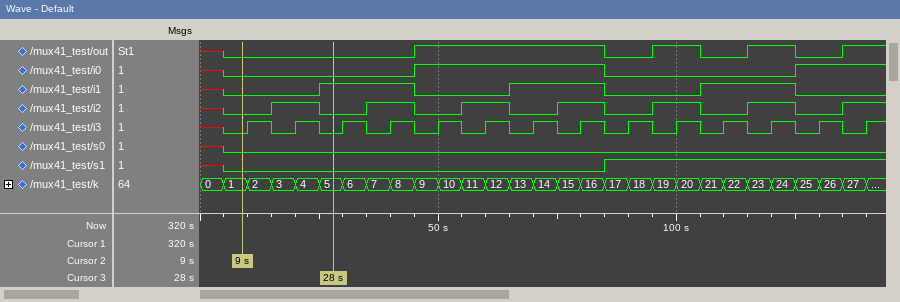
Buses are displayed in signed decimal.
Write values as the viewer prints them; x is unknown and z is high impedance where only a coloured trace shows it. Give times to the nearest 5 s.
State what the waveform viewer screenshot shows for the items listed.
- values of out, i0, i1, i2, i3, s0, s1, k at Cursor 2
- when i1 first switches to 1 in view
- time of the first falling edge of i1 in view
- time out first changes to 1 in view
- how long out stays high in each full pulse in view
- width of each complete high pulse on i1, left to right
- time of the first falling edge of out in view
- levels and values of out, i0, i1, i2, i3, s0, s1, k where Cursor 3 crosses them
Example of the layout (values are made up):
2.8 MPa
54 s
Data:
out=0, i0=0, i1=0, i2=0, i3=0, s0=0, s1=0, k=1
25 s
45 s
45 s
40 s, 10 s, 10 s
20 s, 20 s, 20 s
85 s
out=0, i0=0, i1=1, i2=0, i3=0, s0=0, s1=0, k=5
